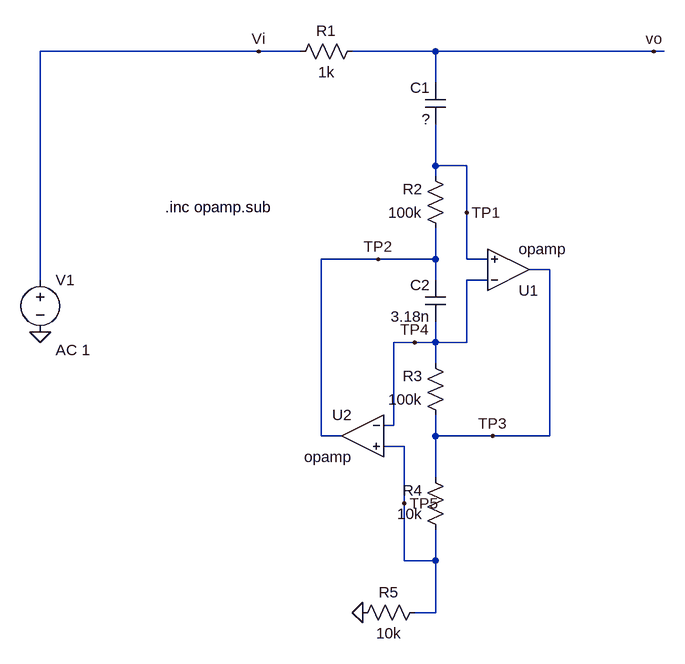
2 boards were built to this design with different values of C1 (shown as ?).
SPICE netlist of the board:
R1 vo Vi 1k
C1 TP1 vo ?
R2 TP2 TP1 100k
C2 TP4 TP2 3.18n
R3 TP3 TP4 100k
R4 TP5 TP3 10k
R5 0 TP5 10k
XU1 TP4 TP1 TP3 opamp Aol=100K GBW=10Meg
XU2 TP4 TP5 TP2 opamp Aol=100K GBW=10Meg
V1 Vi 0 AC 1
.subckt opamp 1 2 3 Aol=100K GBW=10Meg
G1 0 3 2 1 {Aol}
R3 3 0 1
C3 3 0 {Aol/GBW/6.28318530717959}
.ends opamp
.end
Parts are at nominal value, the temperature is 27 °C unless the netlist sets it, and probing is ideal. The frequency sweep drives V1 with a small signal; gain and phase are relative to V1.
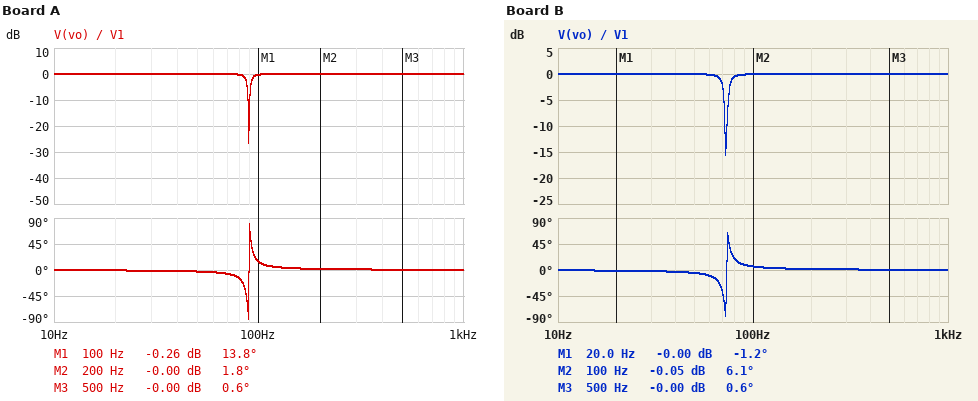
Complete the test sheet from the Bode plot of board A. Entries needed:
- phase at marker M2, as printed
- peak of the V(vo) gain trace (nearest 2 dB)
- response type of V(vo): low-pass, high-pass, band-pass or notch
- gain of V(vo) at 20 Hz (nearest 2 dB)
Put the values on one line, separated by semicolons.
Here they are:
1.8 deg; 0 dB; notch; 0 dB
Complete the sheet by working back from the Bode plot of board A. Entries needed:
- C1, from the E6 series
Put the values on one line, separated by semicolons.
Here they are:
100 nF
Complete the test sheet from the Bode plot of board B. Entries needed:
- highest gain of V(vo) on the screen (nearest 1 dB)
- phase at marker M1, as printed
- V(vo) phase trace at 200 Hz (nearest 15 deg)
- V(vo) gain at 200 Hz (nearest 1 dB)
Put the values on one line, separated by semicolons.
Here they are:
0 dB; -1.2 deg; 0 deg; 0 dB
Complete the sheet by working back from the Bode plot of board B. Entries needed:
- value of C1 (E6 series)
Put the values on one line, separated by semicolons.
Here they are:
150 nF
